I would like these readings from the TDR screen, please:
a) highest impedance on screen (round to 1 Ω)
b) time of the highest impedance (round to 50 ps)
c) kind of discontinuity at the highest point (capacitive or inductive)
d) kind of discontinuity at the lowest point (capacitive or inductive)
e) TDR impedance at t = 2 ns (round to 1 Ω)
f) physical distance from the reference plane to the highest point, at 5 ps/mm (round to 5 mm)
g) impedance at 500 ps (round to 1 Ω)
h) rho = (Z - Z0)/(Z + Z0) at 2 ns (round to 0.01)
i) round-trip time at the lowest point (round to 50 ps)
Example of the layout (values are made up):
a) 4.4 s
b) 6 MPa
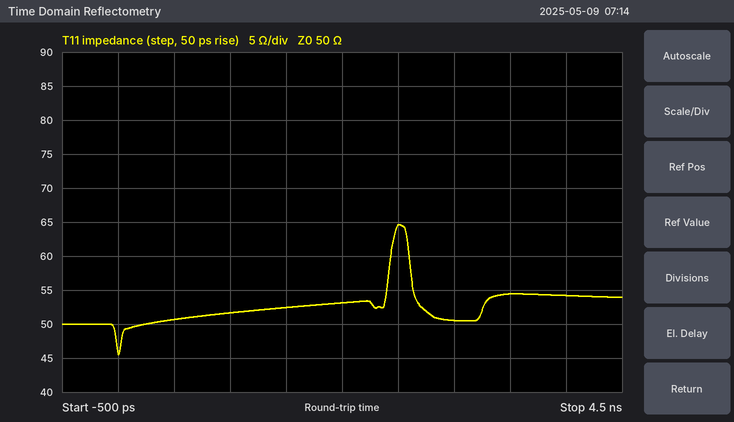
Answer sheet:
a) 65 Ω
b) 2.50 ns
c) inductive
d) capacitive
e) 53 Ω
f) 250 mm
g) 51 Ω
h) +0.03
i) 0 ps
